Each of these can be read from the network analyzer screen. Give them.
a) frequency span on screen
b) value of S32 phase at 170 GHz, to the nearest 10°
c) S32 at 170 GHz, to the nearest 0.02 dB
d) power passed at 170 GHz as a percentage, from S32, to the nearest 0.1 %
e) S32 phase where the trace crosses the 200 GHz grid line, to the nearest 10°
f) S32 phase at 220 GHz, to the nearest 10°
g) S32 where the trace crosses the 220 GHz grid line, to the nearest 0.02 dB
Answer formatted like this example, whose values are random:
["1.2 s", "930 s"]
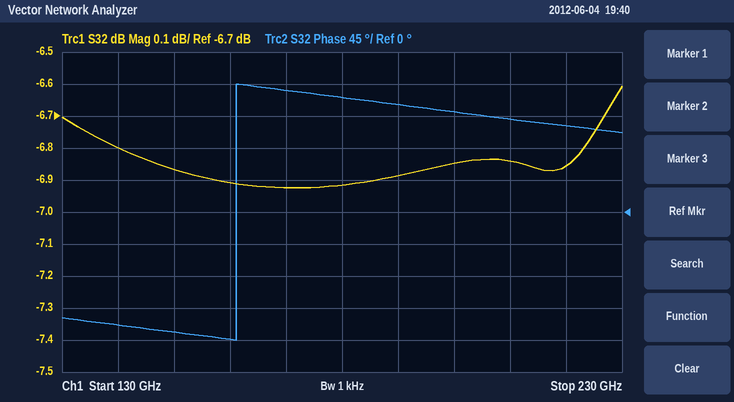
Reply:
["100 GHz", "170°", "-6.92 dB", "20.3 %", "140°", "120°", "-6.86 dB"]
